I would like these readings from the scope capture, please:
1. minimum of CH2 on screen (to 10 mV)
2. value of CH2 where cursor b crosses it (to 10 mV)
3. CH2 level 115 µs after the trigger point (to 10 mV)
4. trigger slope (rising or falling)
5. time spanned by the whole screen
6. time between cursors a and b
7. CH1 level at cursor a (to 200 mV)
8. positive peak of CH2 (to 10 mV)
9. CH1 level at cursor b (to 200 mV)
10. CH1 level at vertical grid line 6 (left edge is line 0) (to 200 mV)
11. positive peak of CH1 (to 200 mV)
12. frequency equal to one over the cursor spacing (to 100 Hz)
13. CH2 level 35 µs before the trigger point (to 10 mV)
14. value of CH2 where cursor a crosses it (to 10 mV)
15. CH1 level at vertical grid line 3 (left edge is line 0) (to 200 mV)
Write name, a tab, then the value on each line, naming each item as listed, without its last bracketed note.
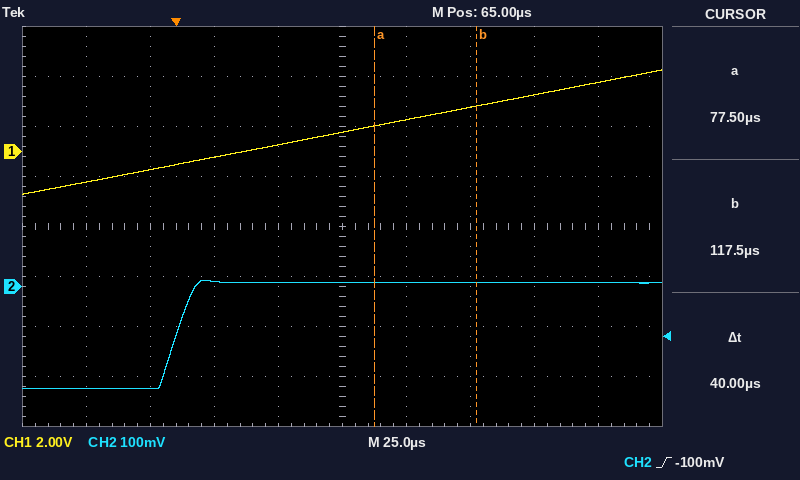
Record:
minimum of CH2 on screen	-200 mV
value of CH2 where cursor b crosses it	10 mV
CH2 level 115 µs after the trigger point	10 mV
trigger slope	rising
time spanned by the whole screen	250 µs
time between cursors a and b	40 µs
CH1 level at cursor a	1.0 V
positive peak of CH2	10 mV
CH1 level at cursor b	1.8 V
CH1 level at vertical grid line 6 (left edge is line 0)	1.2 V
positive peak of CH1	3.2 V
frequency equal to one over the cursor spacing	25.0 kHz
CH2 level 35 µs before the trigger point	-200 mV
value of CH2 where cursor a crosses it	10 mV
CH1 level at vertical grid line 3 (left edge is line 0)	-200 mV
